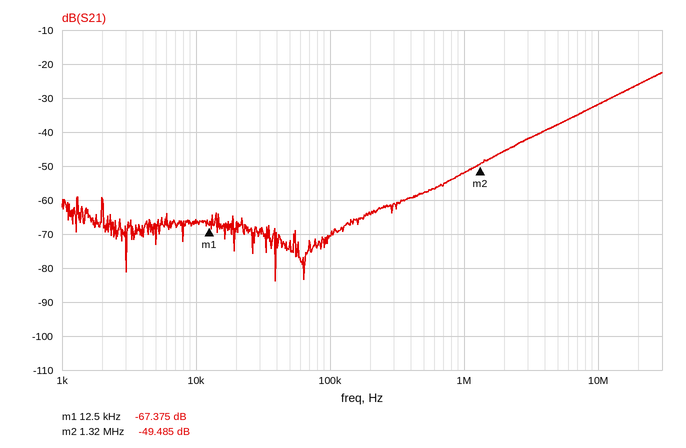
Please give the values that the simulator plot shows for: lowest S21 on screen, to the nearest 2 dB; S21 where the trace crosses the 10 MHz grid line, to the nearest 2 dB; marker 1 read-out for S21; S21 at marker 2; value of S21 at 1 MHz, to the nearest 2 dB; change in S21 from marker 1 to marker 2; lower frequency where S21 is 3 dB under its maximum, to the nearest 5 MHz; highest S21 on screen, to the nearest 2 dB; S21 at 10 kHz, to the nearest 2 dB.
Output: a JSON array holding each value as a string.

["-84 dB", "-32 dB", "-67.375 dB", "-49.485 dB", "-52 dB", "17.890 dB", "20 MHz", "-22 dB", "-66 dB"]
